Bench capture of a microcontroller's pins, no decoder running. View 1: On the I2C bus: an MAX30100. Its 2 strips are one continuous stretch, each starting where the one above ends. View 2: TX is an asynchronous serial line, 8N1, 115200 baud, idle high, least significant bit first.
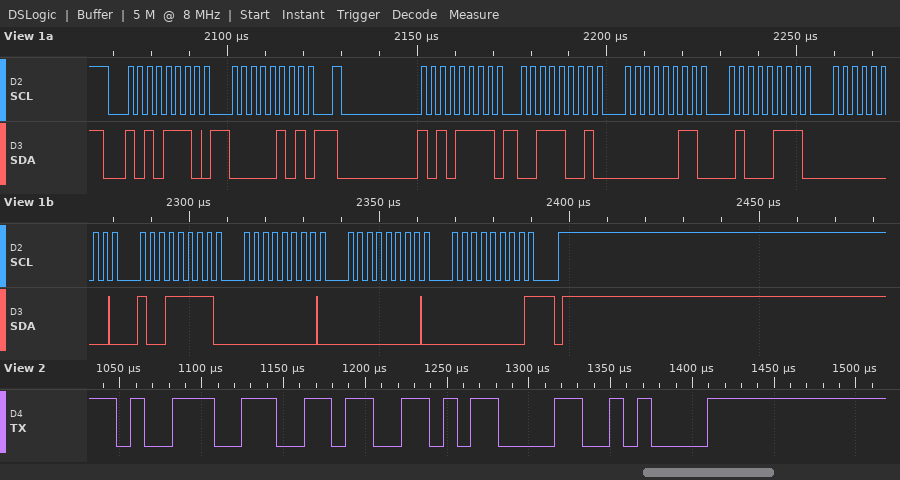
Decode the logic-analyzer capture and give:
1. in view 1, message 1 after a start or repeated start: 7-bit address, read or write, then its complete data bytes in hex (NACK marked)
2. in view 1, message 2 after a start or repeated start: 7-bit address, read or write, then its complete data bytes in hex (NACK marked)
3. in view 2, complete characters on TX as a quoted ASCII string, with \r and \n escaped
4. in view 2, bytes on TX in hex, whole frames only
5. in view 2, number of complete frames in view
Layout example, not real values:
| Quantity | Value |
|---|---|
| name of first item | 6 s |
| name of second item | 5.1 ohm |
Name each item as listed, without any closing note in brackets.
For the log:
| Quantity | Value |
|---|---|
| in view 1, message 1 after a start or repeated start: 7-bit address, read or write, then its complete data bytes in hex | 0x57 write: 05 |
| in view 1, message 2 after a start or repeated start: 7-bit address, read or write, then its complete data bytes in hex | 0x57 read: 39 03 47 00 9F 00 00 00 NACK |
| in view 2, complete characters on TX as a quoted ASCII string, with \r and \n escaped | "96\r\n" |
| in view 2, bytes on TX in hex, whole frames only | 0x39 0x36 0x0D 0x0A |
| in view 2, number of complete frames in view | 4 |
